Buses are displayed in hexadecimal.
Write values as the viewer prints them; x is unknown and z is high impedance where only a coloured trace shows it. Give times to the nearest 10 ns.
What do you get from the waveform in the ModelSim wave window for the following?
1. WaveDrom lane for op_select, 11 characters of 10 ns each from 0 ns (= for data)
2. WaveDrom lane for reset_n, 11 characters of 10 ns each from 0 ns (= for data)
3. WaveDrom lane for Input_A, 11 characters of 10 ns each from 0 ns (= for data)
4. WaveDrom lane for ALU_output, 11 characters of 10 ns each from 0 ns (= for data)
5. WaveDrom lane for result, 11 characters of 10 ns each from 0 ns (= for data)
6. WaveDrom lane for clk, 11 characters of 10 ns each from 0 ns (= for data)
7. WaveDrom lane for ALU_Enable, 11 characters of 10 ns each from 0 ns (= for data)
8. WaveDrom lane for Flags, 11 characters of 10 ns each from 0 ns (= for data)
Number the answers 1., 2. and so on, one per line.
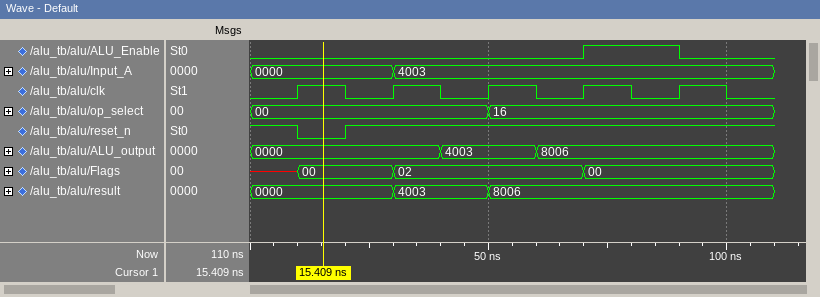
1. {name: 'op_select', wave: '=....=.....', data: '00 16'}
2. {name: 'reset_n', wave: '101........'}
3. {name: 'Input_A', wave: '=..=.......', data: '0000 4003'}
4. {name: 'ALU_output', wave: '=...=.=....', data: '0000 4003 8006'}
5. {name: 'result', wave: '=..=.=.....', data: '0000 4003 8006'}
6. {name: 'clk', wave: '01010101010'}
7. {name: 'ALU_Enable', wave: '0......1.0.'}
8. {name: 'Flags', wave: 'x=.=...=...', data: '00 02 00'}
